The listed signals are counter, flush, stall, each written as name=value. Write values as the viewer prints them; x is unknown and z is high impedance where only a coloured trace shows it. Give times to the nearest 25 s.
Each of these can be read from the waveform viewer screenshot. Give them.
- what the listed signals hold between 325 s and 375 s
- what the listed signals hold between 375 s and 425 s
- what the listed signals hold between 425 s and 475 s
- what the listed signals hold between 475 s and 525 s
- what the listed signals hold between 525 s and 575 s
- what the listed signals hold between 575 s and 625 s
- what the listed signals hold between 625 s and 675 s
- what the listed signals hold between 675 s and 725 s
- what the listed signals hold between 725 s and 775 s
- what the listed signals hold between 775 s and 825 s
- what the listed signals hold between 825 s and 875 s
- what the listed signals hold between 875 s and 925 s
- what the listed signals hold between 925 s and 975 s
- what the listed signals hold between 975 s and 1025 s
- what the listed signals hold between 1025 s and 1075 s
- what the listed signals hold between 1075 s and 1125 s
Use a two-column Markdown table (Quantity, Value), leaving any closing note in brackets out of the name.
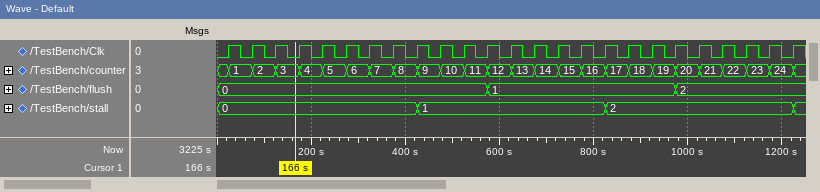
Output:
| Quantity | Value |
|---|---|
| what the listed signals hold between 325 s and 375 s | counter=7, flush=0, stall=0 |
| what the listed signals hold between 375 s and 425 s | counter=8, flush=0, stall=0 |
| what the listed signals hold between 425 s and 475 s | counter=9, flush=0, stall=1 |
| what the listed signals hold between 475 s and 525 s | counter=10, flush=0, stall=1 |
| what the listed signals hold between 525 s and 575 s | counter=11, flush=0, stall=1 |
| what the listed signals hold between 575 s and 625 s | counter=12, flush=1, stall=1 |
| what the listed signals hold between 625 s and 675 s | counter=13, flush=1, stall=1 |
| what the listed signals hold between 675 s and 725 s | counter=14, flush=1, stall=1 |
| what the listed signals hold between 725 s and 775 s | counter=15, flush=1, stall=1 |
| what the listed signals hold between 775 s and 825 s | counter=16, flush=1, stall=1 |
| what the listed signals hold between 825 s and 875 s | counter=17, flush=1, stall=2 |
| what the listed signals hold between 875 s and 925 s | counter=18, flush=1, stall=2 |
| what the listed signals hold between 925 s and 975 s | counter=19, flush=1, stall=2 |
| what the listed signals hold between 975 s and 1025 s | counter=20, flush=2, stall=2 |
| what the listed signals hold between 1025 s and 1075 s | counter=21, flush=2, stall=2 |
| what the listed signals hold between 1075 s and 1125 s | counter=22, flush=2, stall=2 |
